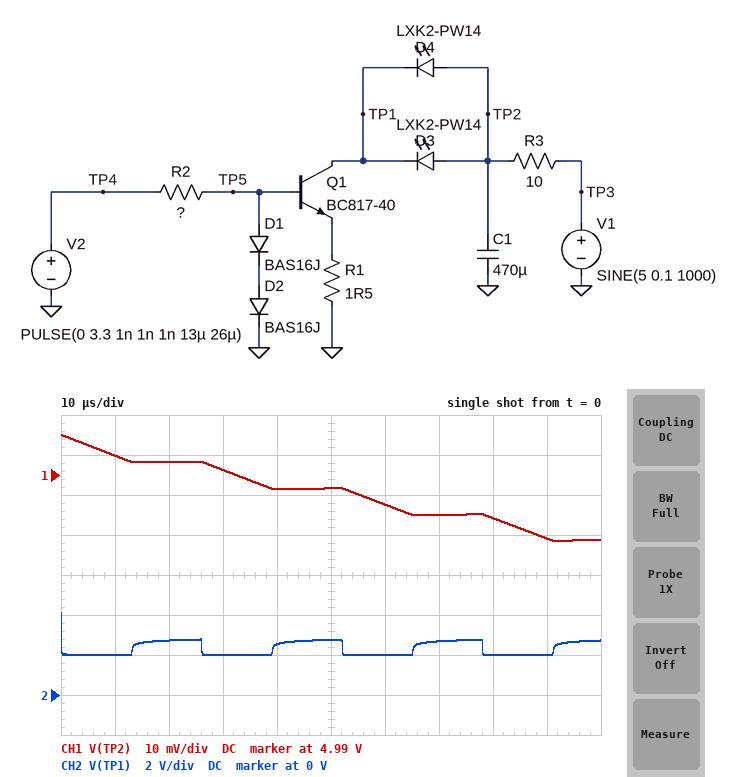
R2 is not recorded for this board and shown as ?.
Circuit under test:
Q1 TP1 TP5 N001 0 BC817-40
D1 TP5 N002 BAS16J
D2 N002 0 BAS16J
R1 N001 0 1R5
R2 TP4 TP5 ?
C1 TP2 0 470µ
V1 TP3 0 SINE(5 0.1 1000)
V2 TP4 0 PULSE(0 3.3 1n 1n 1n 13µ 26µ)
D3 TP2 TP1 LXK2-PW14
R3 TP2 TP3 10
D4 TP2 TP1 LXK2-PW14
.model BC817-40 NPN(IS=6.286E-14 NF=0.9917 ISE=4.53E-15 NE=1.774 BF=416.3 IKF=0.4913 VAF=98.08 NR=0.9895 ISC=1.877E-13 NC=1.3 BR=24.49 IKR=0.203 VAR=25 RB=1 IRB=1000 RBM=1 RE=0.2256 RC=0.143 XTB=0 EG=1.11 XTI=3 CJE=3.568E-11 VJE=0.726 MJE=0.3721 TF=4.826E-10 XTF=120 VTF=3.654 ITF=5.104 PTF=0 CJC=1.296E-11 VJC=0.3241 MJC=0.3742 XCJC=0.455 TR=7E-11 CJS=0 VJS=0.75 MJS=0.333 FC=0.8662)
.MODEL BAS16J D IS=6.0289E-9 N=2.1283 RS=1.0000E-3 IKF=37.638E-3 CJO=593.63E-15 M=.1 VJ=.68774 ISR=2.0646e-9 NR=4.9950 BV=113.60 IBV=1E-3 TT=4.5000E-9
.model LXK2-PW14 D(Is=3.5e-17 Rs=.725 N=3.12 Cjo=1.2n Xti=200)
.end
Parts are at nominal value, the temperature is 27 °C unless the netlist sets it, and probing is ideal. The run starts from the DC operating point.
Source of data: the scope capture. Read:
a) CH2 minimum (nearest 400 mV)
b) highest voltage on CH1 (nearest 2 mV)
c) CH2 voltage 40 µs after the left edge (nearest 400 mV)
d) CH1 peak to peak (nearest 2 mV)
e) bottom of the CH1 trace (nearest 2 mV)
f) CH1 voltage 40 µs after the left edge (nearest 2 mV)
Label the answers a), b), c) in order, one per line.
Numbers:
a) 2.0 V
b) 5.000 V
c) 2.4 V
d) 26 mV
e) 4.974 V
f) 4.986 V
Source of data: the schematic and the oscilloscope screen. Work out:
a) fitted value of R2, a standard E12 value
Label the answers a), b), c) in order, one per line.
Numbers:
a) 1.8 kΩ
